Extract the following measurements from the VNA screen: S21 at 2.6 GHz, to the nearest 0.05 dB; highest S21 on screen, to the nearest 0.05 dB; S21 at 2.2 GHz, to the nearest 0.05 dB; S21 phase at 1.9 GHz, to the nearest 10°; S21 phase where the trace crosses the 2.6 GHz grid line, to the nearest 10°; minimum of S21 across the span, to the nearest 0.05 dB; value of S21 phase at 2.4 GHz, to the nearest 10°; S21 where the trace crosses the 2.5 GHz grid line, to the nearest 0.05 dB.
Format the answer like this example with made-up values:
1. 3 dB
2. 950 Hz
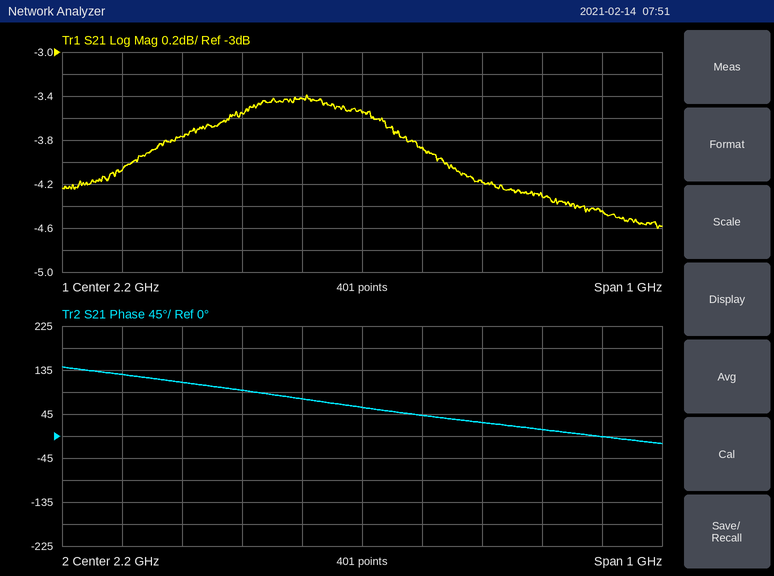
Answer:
1. -4.45 dB
2. -3.40 dB
3. -3.55 dB
4. 110°
5. 0°
6. -4.60 dB
7. 30°
8. -4.30 dB
